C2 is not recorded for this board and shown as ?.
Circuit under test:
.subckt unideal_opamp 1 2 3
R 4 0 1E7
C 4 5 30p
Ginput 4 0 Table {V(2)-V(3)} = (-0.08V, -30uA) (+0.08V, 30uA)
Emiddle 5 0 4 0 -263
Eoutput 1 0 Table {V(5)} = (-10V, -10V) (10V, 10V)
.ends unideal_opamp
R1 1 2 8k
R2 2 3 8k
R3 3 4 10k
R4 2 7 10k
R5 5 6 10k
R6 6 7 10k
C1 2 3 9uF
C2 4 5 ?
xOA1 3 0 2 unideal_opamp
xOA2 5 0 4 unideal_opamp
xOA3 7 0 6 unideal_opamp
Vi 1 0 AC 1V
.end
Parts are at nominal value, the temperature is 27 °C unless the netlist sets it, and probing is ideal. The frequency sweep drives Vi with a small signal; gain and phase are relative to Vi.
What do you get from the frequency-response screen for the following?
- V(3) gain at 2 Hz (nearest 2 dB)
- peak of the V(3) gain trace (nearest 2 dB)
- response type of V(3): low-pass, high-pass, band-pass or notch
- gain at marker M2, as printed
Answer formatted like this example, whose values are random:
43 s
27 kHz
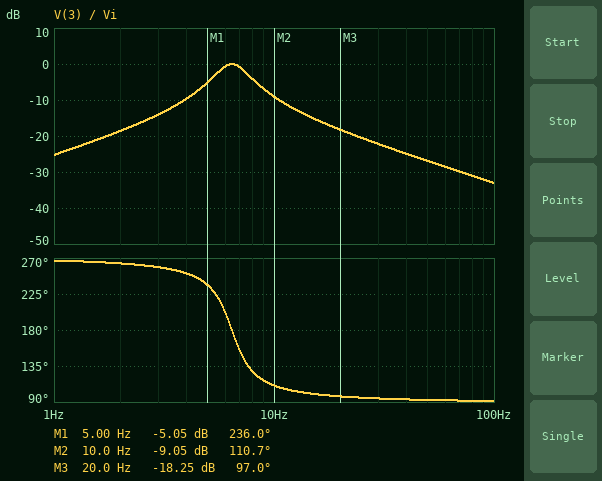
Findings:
-18 dB
0 dB
band-pass
-9.05 dB
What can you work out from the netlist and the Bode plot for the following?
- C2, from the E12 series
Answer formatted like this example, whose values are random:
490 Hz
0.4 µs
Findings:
680 nF
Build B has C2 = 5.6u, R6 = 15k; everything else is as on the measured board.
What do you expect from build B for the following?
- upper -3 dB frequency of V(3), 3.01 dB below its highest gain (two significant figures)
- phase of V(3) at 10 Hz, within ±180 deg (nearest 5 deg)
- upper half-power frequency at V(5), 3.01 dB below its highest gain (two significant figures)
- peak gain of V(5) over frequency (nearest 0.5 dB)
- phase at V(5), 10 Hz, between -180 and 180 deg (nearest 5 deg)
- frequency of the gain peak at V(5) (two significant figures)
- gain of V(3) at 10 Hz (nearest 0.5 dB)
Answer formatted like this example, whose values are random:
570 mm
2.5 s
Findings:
4.1 Hz
105 deg
3.3 Hz
1.0 dB
-165 deg
2.3 Hz
-12.5 dB
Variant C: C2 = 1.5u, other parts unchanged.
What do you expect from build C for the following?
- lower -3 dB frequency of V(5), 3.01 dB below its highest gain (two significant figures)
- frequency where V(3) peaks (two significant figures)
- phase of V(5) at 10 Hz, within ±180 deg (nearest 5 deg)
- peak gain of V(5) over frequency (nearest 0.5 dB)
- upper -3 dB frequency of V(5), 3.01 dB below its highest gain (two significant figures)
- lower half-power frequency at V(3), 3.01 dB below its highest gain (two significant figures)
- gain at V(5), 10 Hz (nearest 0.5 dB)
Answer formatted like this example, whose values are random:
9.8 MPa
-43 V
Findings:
2.7 Hz
4.3 Hz
-165 deg
8.0 dB
5.1 Hz
3.4 Hz
-11.0 dB
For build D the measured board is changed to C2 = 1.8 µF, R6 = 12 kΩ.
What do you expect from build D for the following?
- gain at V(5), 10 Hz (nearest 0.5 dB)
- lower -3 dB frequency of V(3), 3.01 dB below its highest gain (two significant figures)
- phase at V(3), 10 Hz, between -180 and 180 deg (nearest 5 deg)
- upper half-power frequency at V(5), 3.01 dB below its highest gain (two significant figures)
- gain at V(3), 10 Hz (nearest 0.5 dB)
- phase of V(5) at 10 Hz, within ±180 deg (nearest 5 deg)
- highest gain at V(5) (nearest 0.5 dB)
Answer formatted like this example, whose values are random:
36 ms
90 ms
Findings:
-12.5 dB
3.4 Hz
105 deg
5.1 Hz
-11.5 dB
-165 deg
6.5 dB
